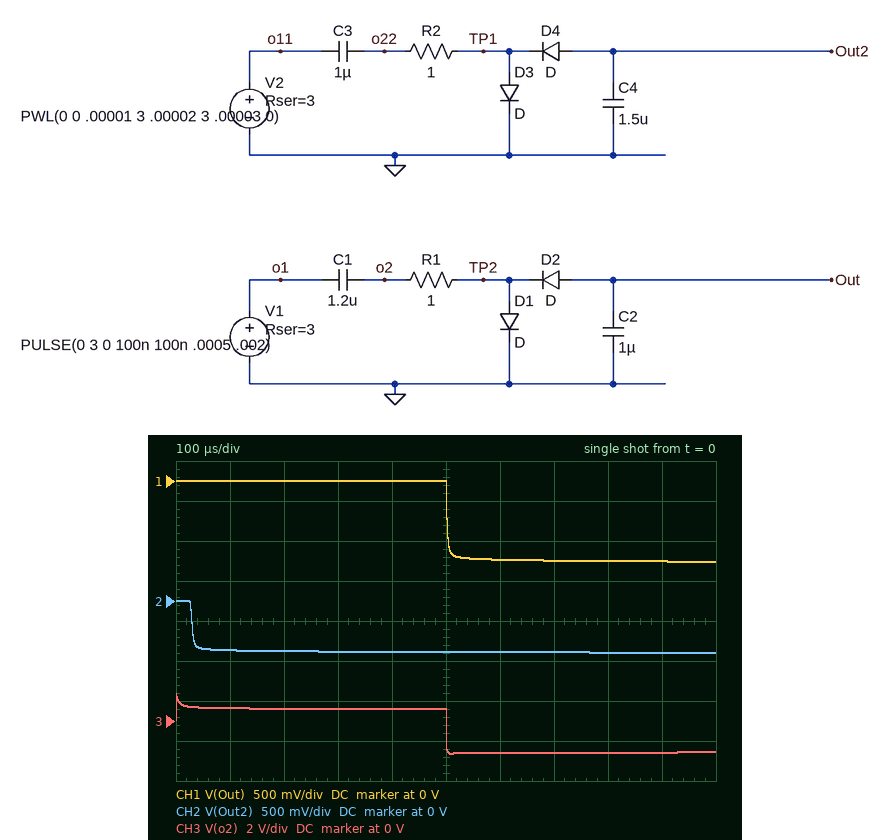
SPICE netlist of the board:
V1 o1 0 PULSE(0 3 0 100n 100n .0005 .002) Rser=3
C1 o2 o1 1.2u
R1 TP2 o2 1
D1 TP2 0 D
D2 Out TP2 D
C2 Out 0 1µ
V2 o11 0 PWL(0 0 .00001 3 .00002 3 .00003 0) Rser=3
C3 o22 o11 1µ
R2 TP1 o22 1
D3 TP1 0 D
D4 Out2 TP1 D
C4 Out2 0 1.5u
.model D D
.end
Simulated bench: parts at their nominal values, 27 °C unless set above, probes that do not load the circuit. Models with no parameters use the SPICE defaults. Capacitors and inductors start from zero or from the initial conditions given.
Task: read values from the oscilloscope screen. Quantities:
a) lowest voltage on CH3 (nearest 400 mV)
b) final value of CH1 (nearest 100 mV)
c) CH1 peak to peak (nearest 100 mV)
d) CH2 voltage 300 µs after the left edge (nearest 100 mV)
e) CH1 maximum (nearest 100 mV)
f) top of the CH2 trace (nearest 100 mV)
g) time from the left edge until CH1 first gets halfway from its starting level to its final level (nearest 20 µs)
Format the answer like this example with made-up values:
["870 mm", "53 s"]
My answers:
["-1.6 V", "-1.0 V", "1.0 V", "-600 mV", "0 V", "0 V", "500 µs"]
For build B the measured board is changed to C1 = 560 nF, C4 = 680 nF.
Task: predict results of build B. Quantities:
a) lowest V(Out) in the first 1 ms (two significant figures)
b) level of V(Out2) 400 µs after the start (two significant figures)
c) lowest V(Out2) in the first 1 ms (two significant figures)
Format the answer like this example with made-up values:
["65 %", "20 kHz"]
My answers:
["-680 mV", "-950 mV", "-970 mV"]
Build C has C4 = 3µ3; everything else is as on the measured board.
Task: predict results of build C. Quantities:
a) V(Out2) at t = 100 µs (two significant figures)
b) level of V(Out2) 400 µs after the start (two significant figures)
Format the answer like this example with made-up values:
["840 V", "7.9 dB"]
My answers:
["-360 mV", "-370 mV"]
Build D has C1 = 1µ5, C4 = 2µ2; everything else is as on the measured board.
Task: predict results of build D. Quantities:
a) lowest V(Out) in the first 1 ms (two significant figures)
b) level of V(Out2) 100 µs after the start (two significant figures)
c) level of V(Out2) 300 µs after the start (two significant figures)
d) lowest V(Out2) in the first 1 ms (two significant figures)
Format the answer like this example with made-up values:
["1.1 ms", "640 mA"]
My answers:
["-1.1 V", "-480 mV", "-490 mV", "-500 mV"]
